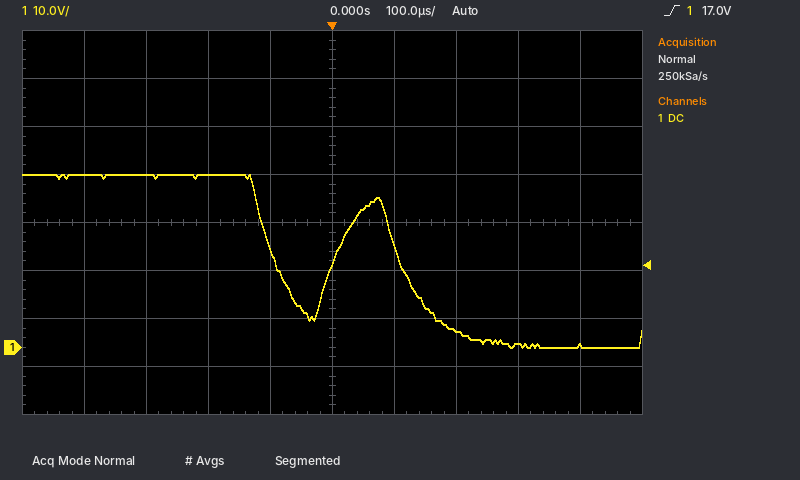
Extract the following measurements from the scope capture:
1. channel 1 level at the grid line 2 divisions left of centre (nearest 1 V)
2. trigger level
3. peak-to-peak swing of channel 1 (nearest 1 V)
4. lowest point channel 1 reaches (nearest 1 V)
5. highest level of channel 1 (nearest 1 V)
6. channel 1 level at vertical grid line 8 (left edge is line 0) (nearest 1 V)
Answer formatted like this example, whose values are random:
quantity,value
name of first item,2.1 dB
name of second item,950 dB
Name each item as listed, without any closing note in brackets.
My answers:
quantity,value
channel 1 level at the grid line 2 divisions left of centre,36 V
trigger level,17.0 V
peak-to-peak swing of channel 1,36 V
lowest point channel 1 reaches,0 V
highest level of channel 1,36 V
channel 1 level at vertical grid line 8 (left edge is line 0),1 V
